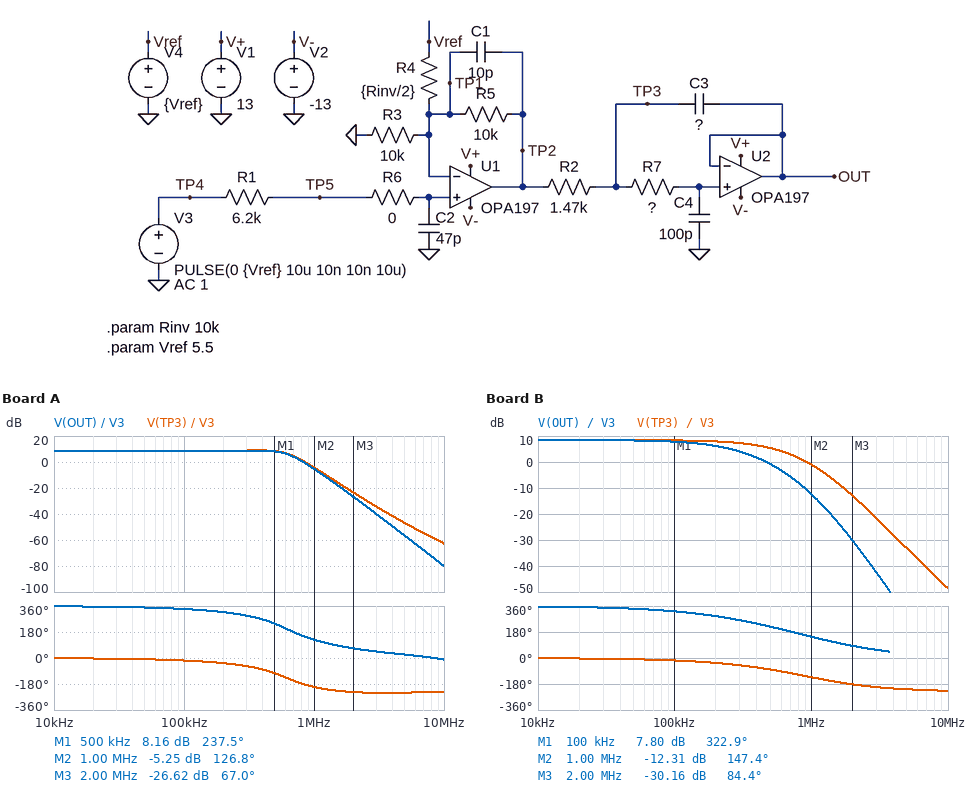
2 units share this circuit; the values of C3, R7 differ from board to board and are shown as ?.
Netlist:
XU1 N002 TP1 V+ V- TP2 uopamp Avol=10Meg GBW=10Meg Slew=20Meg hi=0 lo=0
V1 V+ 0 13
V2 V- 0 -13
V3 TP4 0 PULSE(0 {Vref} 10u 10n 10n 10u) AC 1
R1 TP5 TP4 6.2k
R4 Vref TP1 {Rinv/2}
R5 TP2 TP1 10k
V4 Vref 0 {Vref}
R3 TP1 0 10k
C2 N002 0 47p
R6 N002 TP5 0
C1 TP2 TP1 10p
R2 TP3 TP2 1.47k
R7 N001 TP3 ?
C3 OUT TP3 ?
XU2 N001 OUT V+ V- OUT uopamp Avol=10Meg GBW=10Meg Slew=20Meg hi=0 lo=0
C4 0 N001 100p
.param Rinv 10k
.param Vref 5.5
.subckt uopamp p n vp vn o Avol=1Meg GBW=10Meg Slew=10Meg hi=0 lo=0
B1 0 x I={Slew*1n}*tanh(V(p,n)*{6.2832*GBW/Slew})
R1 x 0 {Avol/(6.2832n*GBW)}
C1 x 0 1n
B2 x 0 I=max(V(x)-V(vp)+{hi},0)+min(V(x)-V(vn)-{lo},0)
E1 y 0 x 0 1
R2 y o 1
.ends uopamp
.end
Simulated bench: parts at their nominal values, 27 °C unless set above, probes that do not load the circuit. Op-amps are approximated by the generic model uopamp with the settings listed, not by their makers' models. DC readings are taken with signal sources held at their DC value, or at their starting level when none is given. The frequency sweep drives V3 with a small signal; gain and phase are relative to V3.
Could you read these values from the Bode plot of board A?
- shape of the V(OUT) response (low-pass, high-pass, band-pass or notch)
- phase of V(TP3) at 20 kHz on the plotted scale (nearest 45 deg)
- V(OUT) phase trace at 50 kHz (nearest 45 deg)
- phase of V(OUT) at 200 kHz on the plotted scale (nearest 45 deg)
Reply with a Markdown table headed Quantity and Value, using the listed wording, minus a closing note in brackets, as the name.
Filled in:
| Quantity | Value |
|---|---|
| shape of the V(OUT) response | low-pass |
| phase of V(TP3) at 20 kHz on the plotted scale | 0 deg |
| V(OUT) phase trace at 50 kHz | 360 deg |
| phase of V(OUT) at 200 kHz on the plotted scale | 315 deg |
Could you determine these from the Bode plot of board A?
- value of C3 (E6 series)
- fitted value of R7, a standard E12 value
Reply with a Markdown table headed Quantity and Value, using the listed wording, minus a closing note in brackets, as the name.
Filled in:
| Quantity | Value |
|---|---|
| value of C3 | 470 pF |
| fitted value of R7, a standard E12 value | 820 Ω |
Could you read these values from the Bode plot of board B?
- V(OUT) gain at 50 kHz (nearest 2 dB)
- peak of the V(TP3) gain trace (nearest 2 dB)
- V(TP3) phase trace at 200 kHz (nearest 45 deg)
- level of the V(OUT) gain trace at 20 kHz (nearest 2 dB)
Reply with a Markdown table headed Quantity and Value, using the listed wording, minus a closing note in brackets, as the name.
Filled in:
| Quantity | Value |
|---|---|
| V(OUT) gain at 50 kHz | 8 dB |
| peak of the V(TP3) gain trace | 8 dB |
| V(TP3) phase trace at 200 kHz | -45 deg |
| level of the V(OUT) gain trace at 20 kHz | 8 dB |
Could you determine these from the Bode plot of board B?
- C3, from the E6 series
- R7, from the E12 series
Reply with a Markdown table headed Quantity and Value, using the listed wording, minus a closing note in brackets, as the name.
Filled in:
| Quantity | Value |
|---|---|
| C3, from the E6 series | 100 pF |
| R7, from the E12 series | 5.6 kΩ |
